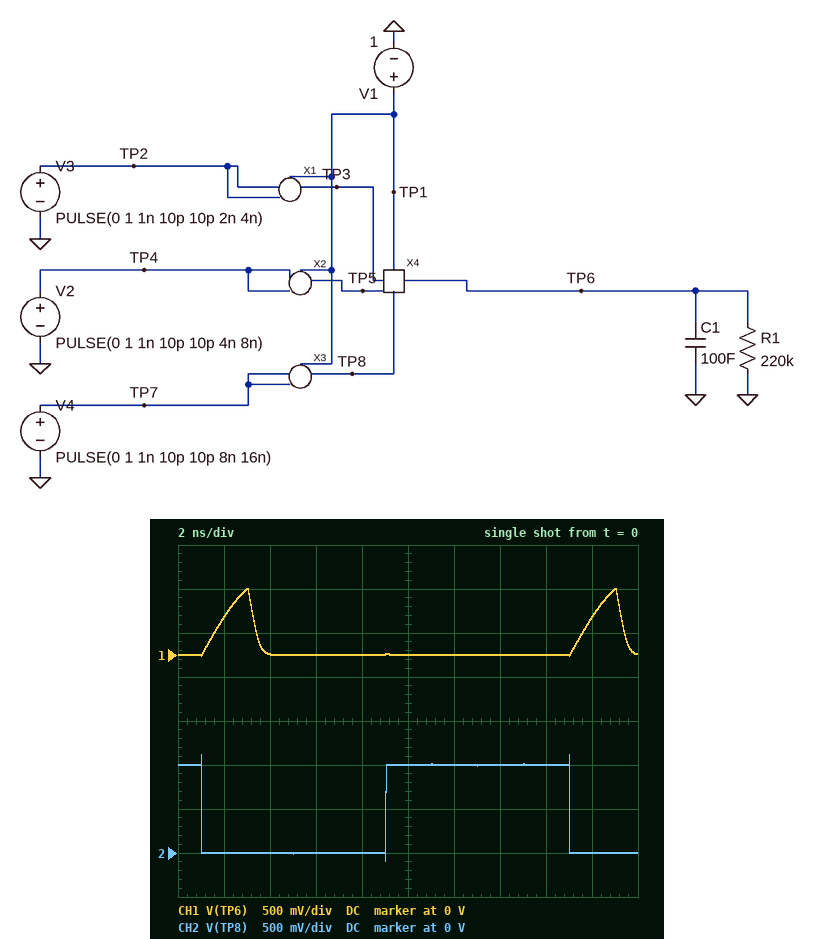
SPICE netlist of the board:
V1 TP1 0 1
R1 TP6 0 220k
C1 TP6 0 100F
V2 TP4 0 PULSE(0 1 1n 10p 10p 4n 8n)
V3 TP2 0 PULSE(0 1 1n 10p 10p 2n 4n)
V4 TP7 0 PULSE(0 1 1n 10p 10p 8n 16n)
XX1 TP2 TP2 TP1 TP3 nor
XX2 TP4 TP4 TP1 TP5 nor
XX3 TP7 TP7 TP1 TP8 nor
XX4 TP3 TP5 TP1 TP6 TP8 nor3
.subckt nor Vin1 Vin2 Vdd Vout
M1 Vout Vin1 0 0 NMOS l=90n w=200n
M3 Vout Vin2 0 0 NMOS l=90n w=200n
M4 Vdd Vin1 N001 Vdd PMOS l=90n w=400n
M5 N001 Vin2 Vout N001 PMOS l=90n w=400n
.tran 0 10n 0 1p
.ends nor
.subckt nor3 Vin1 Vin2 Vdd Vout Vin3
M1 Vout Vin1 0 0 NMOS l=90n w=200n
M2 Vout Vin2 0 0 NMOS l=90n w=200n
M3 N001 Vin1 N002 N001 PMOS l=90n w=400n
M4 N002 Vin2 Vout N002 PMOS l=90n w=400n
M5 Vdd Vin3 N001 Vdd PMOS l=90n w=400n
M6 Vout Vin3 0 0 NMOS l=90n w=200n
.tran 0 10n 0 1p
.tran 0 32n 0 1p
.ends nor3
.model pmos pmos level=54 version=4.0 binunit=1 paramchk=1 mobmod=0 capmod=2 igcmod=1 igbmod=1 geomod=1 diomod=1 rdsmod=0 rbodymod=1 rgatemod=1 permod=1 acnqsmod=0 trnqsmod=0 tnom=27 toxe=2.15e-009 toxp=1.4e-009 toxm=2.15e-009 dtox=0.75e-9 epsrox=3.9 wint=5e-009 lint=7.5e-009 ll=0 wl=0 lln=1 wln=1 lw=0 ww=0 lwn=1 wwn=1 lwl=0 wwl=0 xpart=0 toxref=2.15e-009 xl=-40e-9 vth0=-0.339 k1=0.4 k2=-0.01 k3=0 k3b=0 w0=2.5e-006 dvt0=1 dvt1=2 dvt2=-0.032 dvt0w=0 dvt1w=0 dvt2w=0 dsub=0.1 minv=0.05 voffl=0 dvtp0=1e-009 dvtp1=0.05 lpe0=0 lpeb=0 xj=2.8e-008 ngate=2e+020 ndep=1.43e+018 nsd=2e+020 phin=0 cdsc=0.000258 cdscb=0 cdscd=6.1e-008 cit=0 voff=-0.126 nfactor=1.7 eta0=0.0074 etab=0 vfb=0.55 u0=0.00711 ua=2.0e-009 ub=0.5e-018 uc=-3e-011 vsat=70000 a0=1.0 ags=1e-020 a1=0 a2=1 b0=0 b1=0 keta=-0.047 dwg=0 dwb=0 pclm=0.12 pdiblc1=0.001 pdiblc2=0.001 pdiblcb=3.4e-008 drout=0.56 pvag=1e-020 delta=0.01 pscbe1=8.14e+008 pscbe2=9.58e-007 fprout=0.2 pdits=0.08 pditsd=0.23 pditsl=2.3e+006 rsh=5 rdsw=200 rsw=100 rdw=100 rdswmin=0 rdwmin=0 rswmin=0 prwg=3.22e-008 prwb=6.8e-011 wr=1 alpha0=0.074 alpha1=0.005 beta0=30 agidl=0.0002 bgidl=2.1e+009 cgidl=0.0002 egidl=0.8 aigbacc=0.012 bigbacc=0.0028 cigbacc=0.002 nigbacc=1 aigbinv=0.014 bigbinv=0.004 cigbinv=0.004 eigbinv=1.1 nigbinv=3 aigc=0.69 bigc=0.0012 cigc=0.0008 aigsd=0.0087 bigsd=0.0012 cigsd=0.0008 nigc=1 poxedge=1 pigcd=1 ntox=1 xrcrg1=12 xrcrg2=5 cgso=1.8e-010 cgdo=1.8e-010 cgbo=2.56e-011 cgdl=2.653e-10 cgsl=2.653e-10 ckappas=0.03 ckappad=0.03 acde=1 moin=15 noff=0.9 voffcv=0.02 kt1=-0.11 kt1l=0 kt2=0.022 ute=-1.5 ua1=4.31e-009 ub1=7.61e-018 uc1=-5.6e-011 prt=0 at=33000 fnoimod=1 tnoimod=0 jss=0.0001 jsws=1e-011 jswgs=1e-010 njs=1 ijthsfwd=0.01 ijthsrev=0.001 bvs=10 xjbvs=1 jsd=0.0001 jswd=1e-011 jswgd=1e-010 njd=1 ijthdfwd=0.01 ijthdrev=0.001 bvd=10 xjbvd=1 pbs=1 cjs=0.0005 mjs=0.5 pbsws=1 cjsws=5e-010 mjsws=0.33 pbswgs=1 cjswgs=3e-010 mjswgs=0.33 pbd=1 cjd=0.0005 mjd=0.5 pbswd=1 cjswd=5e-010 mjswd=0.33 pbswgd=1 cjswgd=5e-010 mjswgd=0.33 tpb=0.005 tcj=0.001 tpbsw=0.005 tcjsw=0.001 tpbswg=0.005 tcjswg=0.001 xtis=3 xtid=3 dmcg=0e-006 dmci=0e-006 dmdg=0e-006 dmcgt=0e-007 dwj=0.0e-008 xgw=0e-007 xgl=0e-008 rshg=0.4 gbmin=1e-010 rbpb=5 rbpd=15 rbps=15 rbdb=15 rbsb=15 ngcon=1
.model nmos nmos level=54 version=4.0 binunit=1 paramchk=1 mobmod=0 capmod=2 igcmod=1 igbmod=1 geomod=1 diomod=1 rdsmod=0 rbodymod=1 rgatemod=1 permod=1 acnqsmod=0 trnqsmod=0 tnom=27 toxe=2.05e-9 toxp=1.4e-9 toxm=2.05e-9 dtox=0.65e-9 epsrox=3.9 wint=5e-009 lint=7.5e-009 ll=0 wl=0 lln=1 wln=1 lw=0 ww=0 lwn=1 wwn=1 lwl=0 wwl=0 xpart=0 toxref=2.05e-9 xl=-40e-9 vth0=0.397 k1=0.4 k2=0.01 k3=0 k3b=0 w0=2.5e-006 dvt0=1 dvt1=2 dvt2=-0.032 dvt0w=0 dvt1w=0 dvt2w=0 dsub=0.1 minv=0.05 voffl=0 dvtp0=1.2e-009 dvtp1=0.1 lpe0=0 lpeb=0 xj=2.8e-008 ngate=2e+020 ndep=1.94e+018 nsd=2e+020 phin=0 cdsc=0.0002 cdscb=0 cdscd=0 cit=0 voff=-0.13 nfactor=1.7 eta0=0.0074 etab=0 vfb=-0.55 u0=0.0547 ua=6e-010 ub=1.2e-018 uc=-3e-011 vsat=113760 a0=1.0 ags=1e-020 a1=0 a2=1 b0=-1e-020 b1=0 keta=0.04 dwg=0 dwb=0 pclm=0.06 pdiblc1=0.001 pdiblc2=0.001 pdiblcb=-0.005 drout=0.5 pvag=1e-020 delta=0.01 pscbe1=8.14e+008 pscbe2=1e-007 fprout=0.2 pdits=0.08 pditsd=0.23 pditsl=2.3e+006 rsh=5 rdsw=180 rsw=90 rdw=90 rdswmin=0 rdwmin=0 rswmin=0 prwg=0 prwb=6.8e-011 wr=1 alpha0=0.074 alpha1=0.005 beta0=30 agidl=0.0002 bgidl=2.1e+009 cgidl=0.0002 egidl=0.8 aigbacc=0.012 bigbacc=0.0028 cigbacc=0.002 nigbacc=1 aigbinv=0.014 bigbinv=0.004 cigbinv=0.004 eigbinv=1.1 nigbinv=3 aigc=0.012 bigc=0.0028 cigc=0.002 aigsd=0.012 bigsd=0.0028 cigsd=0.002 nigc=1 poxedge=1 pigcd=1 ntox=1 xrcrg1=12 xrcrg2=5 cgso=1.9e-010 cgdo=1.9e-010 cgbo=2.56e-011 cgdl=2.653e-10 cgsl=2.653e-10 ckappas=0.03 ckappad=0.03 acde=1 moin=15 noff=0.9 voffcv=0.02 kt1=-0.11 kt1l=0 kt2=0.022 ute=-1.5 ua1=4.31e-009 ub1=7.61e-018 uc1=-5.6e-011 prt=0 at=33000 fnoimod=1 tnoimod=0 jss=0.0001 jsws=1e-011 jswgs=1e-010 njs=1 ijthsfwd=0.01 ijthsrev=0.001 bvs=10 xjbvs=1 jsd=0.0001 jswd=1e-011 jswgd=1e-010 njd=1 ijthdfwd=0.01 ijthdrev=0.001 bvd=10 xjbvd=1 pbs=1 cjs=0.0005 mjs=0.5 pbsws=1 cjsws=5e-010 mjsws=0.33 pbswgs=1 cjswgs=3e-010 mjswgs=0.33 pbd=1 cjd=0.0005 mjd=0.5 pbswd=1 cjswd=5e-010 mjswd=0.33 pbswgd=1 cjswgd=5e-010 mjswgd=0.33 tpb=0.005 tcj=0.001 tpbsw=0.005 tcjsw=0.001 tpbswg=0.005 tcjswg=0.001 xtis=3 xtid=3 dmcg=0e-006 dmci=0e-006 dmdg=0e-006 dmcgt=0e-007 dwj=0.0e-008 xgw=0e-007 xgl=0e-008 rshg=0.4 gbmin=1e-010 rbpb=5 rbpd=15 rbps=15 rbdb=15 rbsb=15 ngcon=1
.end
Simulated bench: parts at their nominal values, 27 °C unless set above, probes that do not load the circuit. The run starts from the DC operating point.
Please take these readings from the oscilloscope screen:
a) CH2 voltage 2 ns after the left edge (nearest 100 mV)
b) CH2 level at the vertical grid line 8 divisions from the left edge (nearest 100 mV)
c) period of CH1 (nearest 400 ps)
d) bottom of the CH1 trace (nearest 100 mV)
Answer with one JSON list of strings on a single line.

["0 V", "1.0 V", "16.0 ns", "0 V"]
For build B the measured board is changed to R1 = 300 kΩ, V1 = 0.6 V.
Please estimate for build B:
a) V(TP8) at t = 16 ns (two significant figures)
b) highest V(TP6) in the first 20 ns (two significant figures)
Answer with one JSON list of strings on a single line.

["600 mV", "200 mV"]
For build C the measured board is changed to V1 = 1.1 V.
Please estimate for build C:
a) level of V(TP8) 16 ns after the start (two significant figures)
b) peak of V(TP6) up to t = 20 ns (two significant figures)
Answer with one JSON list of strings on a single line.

["1.1 V", "880 mV"]
